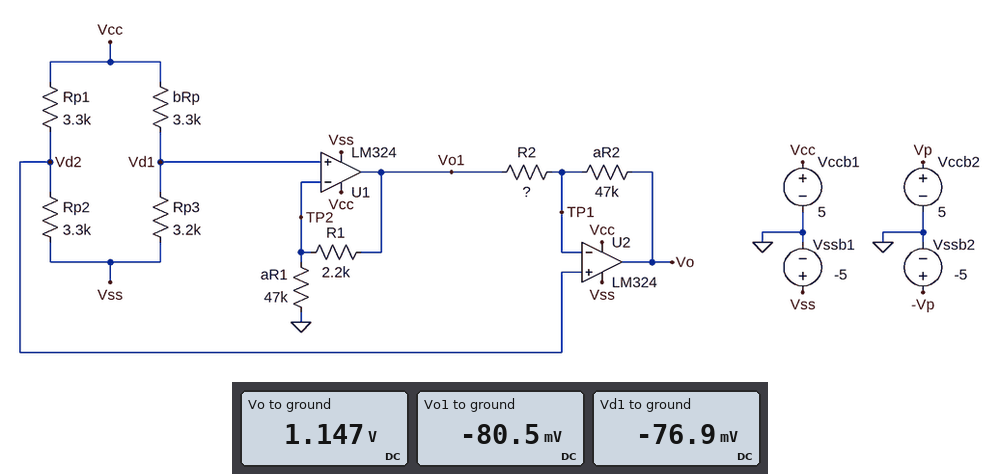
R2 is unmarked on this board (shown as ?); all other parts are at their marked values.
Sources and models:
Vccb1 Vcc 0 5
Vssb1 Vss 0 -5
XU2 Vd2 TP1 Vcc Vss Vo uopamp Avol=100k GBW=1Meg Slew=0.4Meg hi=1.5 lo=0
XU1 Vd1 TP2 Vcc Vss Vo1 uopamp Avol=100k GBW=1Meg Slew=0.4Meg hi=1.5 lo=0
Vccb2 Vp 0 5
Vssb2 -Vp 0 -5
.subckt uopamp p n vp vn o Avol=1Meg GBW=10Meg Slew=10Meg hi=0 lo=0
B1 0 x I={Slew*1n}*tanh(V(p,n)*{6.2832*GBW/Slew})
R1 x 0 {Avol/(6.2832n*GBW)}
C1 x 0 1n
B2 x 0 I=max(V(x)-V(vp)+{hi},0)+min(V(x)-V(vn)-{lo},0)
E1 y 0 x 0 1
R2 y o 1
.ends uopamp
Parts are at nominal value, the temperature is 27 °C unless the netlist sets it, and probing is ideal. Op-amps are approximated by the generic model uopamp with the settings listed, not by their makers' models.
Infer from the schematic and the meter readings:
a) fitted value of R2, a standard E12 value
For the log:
3.3 kΩ
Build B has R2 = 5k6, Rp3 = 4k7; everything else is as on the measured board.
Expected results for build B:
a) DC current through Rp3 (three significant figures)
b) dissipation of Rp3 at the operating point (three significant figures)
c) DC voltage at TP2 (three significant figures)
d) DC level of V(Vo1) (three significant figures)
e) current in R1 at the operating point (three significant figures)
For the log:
1.25 mA
7.34 mW
875 mV
916 mV
18.6 µA
